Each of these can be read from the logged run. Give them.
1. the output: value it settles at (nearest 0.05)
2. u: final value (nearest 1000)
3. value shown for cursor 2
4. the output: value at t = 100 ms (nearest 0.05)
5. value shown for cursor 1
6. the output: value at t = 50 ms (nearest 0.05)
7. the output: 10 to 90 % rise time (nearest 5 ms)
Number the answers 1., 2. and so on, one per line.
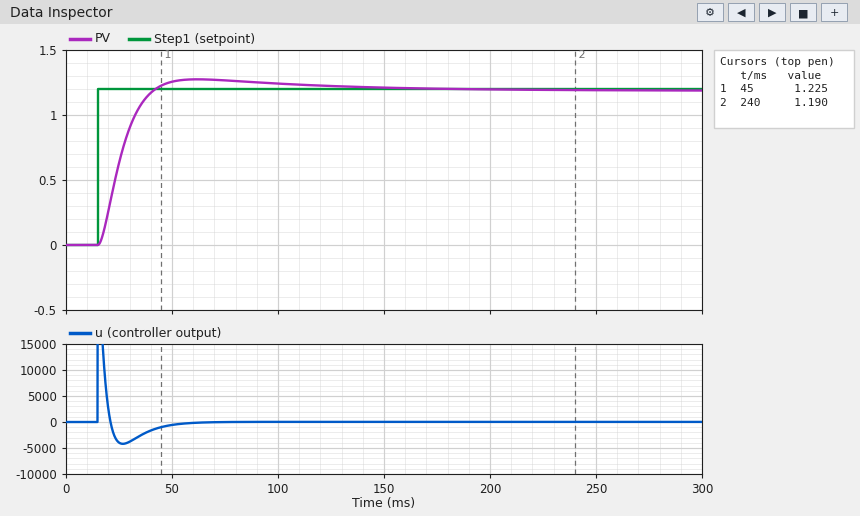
1. 1.20
2. 0
3. 1.190
4. 1.25
5. 1.225
6. 1.25
7. 15 ms
